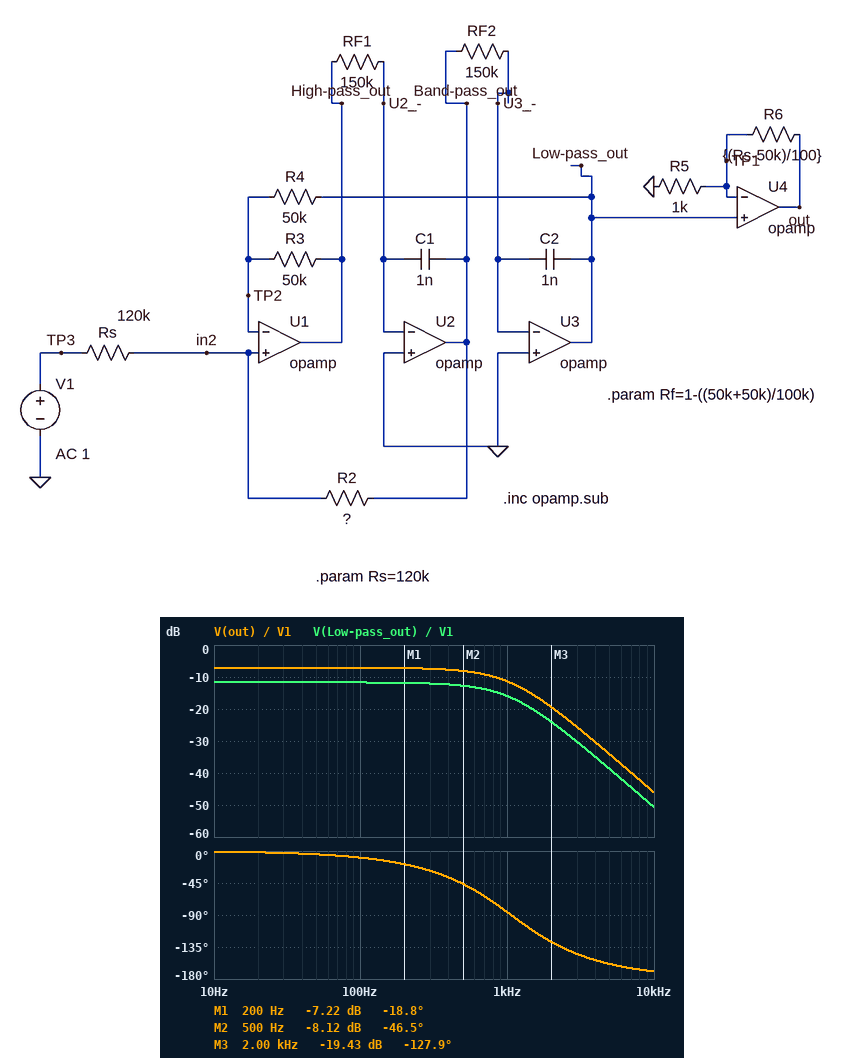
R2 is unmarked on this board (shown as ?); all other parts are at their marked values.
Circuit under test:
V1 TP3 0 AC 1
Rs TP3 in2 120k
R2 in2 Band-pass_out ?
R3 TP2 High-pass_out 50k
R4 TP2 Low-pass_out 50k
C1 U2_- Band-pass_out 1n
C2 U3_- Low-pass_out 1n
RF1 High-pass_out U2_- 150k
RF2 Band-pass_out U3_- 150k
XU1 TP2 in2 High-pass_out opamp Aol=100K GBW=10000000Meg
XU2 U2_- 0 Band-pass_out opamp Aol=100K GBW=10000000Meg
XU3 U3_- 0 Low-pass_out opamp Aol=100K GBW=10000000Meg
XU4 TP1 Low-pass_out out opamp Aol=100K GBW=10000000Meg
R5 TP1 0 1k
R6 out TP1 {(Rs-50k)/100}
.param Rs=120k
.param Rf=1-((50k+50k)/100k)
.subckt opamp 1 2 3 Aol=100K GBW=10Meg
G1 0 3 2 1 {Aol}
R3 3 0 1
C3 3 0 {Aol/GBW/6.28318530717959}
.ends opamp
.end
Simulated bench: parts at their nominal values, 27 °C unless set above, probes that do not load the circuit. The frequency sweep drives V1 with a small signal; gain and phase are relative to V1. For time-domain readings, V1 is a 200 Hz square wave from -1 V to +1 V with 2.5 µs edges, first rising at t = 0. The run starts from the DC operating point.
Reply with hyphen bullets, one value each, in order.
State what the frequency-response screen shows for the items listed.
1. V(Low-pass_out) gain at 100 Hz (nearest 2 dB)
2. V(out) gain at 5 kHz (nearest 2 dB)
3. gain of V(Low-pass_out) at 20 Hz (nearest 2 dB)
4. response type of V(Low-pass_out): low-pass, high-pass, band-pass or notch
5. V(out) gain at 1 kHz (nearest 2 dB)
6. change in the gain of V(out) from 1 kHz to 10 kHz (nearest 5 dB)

- -12 dB
- -34 dB
- -12 dB
- low-pass
- -12 dB
- -35 dB
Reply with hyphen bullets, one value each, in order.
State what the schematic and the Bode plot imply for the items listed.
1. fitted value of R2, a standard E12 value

- 18 kΩ
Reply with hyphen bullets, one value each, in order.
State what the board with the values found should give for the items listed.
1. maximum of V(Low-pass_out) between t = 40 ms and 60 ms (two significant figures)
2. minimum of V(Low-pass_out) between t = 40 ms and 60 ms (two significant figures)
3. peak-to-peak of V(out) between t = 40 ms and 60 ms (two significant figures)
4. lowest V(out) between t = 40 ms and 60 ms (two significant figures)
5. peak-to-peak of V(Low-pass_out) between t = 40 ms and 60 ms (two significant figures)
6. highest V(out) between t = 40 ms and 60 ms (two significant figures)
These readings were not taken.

- 260 mV
- -260 mV
- 890 mV
- -450 mV
- 530 mV
- 450 mV
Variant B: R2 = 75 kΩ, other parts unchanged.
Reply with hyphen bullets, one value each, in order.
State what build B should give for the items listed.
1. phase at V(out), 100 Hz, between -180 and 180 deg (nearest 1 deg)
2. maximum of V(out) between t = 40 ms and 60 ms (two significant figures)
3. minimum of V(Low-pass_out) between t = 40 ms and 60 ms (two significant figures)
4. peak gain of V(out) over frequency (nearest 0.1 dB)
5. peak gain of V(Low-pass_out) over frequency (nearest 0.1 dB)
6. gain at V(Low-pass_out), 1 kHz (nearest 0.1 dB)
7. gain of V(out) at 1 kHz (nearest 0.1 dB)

- -7 deg
- 1.5 V
- -900 mV
- 2.6 dB
- -2.0 dB
- -3.6 dB
- 1.0 dB
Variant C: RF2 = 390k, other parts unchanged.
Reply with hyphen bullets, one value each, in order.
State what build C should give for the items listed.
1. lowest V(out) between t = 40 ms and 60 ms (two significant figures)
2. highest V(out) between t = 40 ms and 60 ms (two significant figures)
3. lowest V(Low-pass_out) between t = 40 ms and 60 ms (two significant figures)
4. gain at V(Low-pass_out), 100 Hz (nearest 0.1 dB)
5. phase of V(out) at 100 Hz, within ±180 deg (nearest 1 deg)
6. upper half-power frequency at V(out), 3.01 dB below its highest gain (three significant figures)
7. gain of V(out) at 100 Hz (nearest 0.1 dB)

- -430 mV
- 430 mV
- -250 mV
- -12.2 dB
- -24 deg
- 268 Hz
- -7.6 dB
